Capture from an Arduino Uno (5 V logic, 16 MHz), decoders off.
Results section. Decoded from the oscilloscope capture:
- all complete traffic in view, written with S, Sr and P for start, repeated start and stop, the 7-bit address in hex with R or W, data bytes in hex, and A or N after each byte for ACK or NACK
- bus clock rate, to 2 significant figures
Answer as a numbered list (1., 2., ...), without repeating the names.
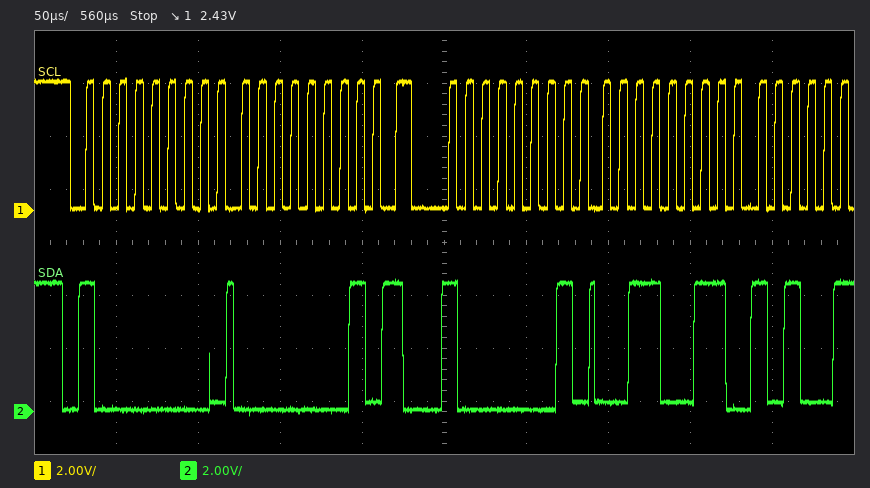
1. S 40W A 01 A Sr 40R A 33 A
2. 100 kHz
